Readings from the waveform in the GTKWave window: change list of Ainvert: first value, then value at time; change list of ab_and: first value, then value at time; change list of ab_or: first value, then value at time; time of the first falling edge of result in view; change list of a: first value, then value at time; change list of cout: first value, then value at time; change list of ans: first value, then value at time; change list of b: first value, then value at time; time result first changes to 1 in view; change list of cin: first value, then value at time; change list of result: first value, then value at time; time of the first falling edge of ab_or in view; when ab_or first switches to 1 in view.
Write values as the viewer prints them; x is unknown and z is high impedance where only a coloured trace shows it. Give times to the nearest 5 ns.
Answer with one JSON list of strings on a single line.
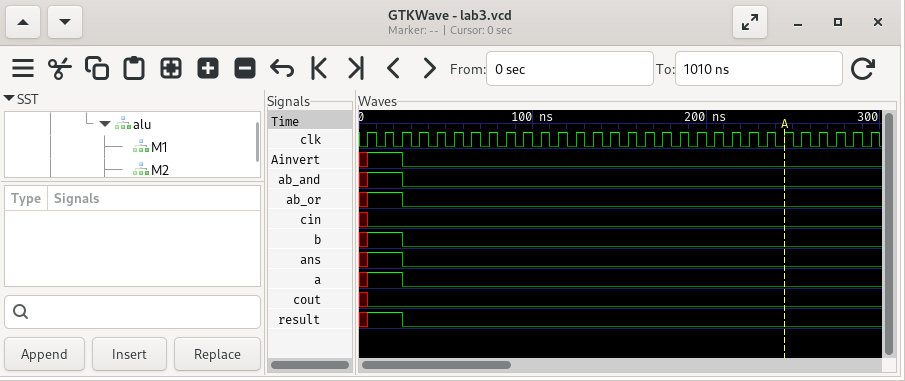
["x, 1 at 5 ns, 0 at 25 ns", "x, 1 at 5 ns, 0 at 25 ns", "x, 1 at 5 ns, 0 at 25 ns", "25 ns", "x, 1 at 5 ns, 0 at 25 ns", "x, 0 at 5 ns", "x, 1 at 5 ns, 0 at 25 ns", "x, 1 at 5 ns, 0 at 25 ns", "5 ns", "x, 0 at 5 ns", "x, 1 at 5 ns, 0 at 25 ns", "25 ns", "5 ns"]
